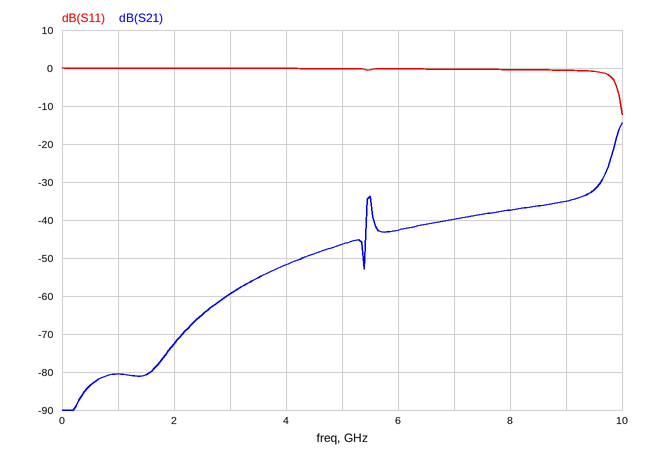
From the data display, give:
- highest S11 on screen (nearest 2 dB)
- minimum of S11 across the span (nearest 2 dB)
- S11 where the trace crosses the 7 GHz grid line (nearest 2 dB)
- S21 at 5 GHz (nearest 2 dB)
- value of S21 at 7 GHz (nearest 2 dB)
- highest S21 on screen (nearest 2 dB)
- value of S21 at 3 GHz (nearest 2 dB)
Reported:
0 dB
-12 dB
0 dB
-46 dB
-40 dB
-14 dB
-60 dB
